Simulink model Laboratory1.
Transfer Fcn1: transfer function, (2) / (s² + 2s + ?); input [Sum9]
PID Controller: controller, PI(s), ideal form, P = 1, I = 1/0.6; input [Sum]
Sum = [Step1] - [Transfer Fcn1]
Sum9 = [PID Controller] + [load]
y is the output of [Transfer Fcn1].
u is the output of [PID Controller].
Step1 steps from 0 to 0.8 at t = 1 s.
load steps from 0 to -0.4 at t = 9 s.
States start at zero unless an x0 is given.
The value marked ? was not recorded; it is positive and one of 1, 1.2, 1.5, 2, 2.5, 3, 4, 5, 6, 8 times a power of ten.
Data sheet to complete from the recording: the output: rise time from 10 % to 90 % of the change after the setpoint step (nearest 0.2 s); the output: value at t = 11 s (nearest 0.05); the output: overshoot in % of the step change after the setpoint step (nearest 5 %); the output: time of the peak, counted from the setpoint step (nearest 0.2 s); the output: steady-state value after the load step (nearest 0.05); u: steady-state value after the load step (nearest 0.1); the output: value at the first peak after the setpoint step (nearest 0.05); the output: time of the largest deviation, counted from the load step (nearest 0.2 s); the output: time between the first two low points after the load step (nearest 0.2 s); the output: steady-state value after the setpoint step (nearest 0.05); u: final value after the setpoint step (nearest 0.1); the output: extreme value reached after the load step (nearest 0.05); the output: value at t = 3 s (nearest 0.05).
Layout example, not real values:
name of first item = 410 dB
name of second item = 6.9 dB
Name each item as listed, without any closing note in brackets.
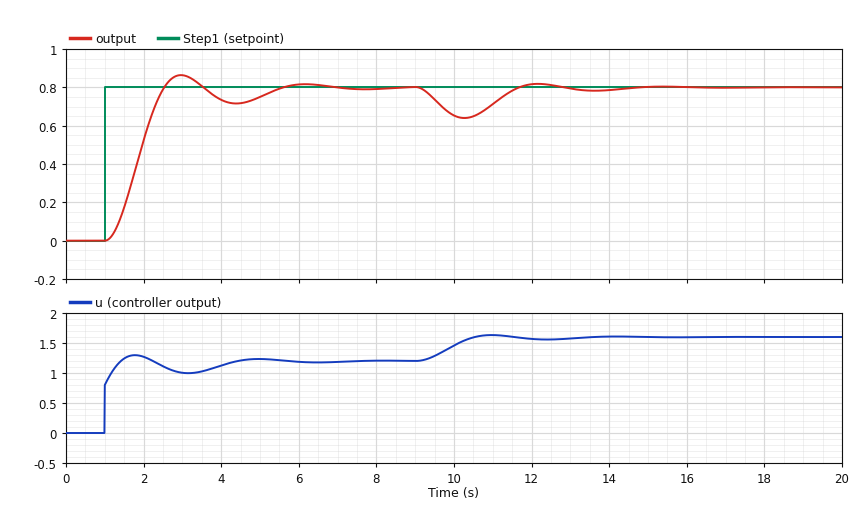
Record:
the output: rise time from 10 % to 90 % of the change after the setpoint step = 1.0 s
the output: value at t = 11 s = 0.70
the output: overshoot in % of the step change after the setpoint step = 10 %
the output: time of the peak, counted from the setpoint step = 2.0 s
the output: steady-state value after the load step = 0.80
u: steady-state value after the load step = 1.6
the output: value at the first peak after the setpoint step = 0.85
the output: time of the largest deviation, counted from the load step = 1.2 s
the output: time between the first two low points after the load step = 3.4 s
the output: steady-state value after the setpoint step = 0.80
u: final value after the setpoint step = 1.2
the output: extreme value reached after the load step = 0.65
the output: value at t = 3 s = 0.85
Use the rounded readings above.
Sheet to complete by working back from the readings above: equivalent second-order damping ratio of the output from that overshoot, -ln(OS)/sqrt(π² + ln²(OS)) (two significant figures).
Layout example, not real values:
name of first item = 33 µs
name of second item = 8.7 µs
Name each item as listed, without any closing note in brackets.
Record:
equivalent second-order damping ratio of the output from that overshoot, -ln(OS)/sqrt(π² + ln²(OS)) = 0.59
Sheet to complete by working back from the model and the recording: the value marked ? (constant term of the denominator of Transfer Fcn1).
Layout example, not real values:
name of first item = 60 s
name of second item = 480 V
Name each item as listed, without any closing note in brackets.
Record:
the value marked ? = 3
